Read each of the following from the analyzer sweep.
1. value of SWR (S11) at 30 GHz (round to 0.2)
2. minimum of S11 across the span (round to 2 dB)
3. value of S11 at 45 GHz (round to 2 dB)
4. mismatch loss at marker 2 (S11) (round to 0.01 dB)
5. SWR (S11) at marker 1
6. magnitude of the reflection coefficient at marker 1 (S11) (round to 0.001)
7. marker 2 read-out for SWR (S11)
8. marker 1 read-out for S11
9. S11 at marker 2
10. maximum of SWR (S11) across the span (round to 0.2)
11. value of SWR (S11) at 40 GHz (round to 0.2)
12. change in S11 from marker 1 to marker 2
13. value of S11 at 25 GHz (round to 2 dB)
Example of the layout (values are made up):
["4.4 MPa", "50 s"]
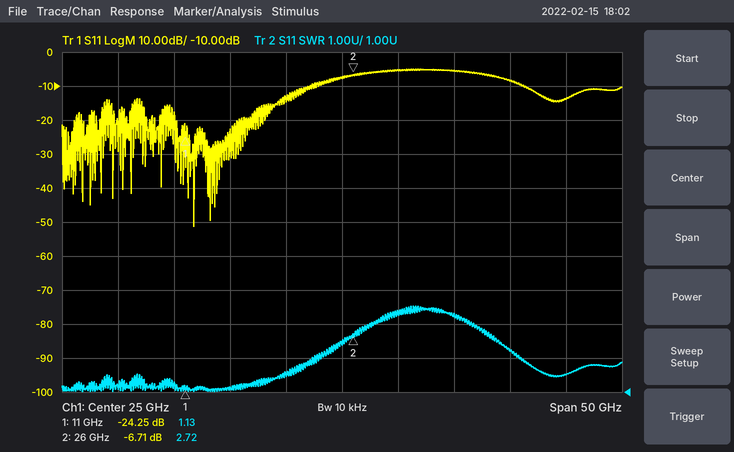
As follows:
["3.4", "-52 dB", "-14 dB", "1.04 dB", "1.13", "0.061", "2.72", "-24.25 dB", "-6.71 dB", "3.6", "2.2", "17.54 dB", "-8 dB"]
